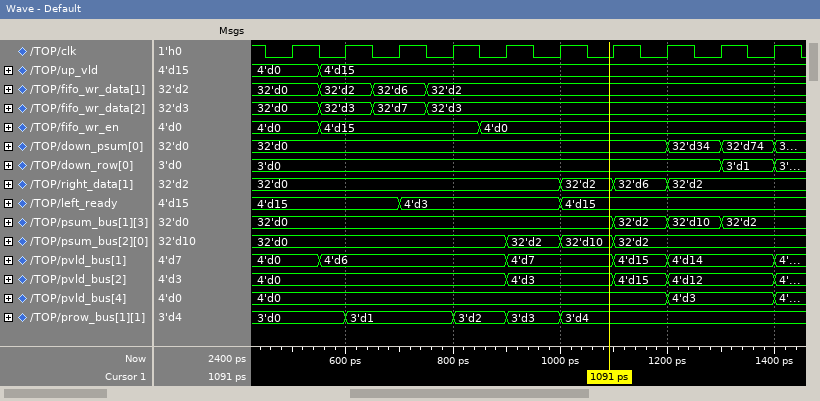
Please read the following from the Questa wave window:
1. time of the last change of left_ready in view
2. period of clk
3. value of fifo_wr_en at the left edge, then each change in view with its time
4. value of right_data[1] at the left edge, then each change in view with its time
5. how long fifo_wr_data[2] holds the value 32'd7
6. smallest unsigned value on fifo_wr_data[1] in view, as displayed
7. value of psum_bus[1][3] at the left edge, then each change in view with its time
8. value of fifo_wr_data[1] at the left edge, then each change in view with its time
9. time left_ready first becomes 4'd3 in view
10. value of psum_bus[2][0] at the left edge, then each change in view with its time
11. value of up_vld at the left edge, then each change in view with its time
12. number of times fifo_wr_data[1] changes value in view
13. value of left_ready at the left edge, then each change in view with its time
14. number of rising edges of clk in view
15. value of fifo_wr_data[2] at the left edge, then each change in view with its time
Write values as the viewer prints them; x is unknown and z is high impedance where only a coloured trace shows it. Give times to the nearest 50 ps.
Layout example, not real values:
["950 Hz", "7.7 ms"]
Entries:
["1000 ps", "100 ps", "4'd0, 4'd15 at 550 ps, 4'd0 at 850 ps", "32'd0, 32'd2 at 1000 ps, 32'd6 at 1100 ps, 32'd2 at 1200 ps", "100 ps", "32'd0", "32'd0, 32'd2 at 1100 ps, 32'd10 at 1200 ps, 32'd2 at 1300 ps", "32'd0, 32'd2 at 550 ps, 32'd6 at 650 ps, 32'd2 at 750 ps", "700 ps", "32'd0, 32'd2 at 900 ps, 32'd10 at 1000 ps, 32'd2 at 1100 ps", "4'd0, 4'd15 at 550 ps", "3", "4'd15, 4'd3 at 700 ps, 4'd15 at 1000 ps", "10", "32'd0, 32'd3 at 550 ps, 32'd7 at 650 ps, 32'd3 at 750 ps"]
